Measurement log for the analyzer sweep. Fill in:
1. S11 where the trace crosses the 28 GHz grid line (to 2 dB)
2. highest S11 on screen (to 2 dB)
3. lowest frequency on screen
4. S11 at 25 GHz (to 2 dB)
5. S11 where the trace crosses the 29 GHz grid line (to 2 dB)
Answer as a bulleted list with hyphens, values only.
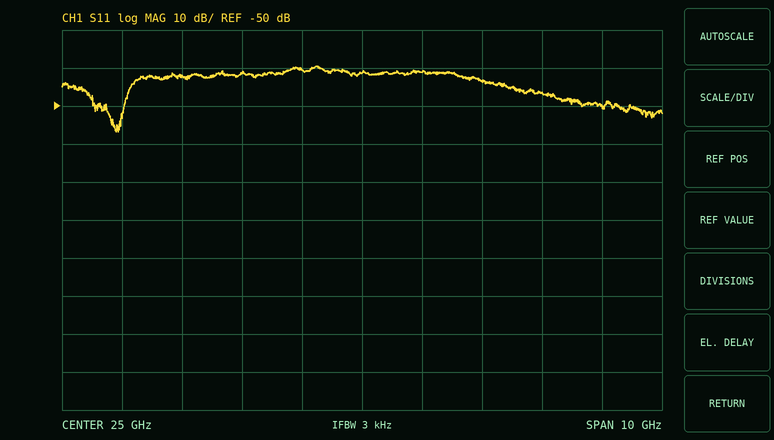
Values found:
- -46 dB
- -40 dB
- 20 GHz
- -42 dB
- -50 dB
